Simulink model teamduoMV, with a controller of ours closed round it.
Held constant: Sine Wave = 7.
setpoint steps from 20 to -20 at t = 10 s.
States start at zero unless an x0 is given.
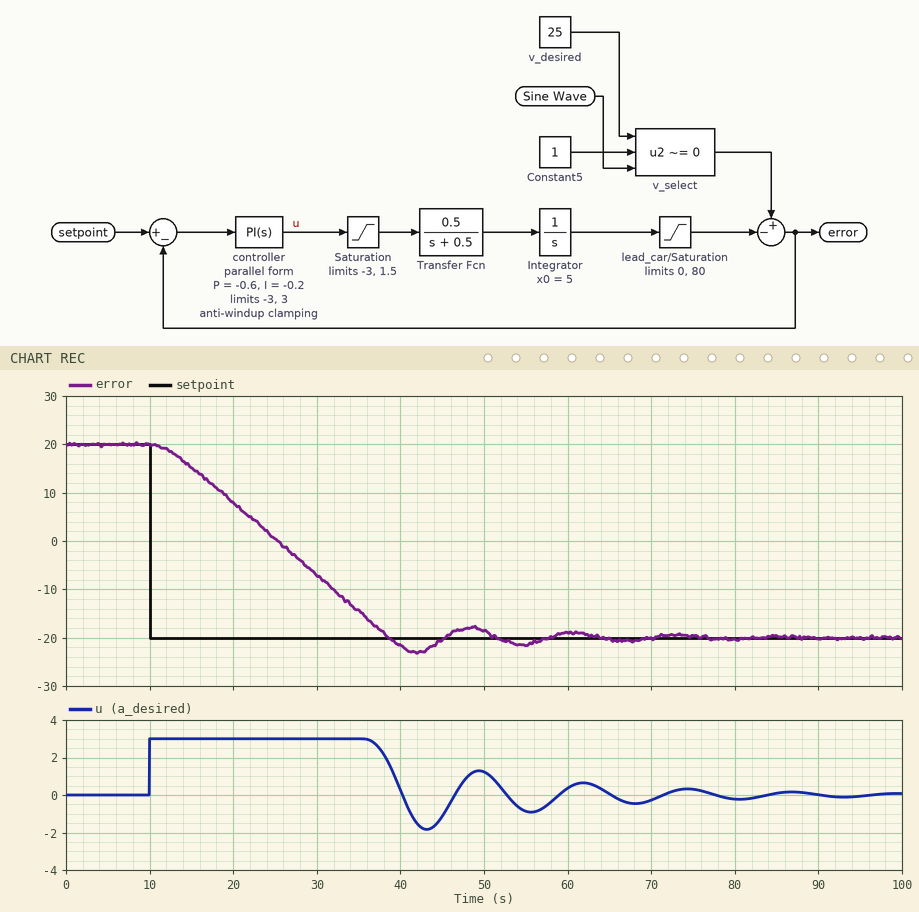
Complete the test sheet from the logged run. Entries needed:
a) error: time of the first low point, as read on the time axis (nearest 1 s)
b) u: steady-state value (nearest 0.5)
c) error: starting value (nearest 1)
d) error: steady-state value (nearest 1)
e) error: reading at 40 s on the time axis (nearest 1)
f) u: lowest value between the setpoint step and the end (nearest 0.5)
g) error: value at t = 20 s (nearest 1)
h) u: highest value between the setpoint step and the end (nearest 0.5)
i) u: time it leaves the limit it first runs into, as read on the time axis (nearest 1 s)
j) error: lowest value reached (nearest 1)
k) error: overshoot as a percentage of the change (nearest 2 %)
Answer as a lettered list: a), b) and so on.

a) 42 s
b) 0.0
c) 20
d) -20
e) -22
f) -2.0
g) 8
h) 3.0
i) 36 s
j) -23
k) 8 %
